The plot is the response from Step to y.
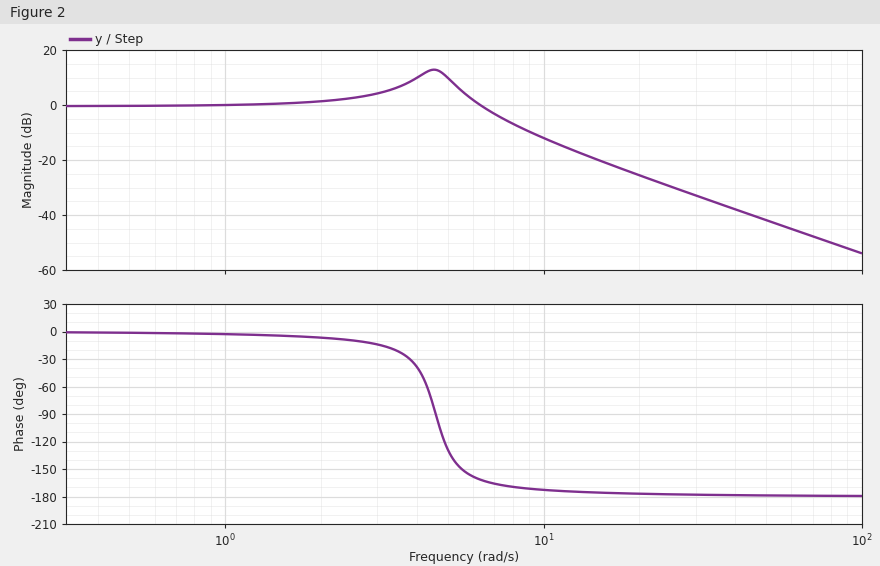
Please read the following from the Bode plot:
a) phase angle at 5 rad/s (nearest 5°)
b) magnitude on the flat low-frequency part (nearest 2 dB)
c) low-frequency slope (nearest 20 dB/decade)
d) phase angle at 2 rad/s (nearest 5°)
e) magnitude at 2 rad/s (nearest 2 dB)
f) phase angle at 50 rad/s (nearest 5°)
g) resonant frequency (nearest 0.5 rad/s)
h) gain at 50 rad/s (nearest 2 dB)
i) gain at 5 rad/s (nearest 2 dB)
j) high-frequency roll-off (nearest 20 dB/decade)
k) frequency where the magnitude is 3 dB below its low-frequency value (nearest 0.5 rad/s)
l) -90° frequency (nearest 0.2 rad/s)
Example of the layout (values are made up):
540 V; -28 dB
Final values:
-130°; 0 dB; 0 dB/decade; -5°; 2 dB; -180°; 4.5 rad/s; -42 dB; 10 dB; -40 dB/decade; 7.0 rad/s; 4.6 rad/s
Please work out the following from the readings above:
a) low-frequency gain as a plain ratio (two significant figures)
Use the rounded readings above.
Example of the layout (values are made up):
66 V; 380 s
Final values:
1.0
